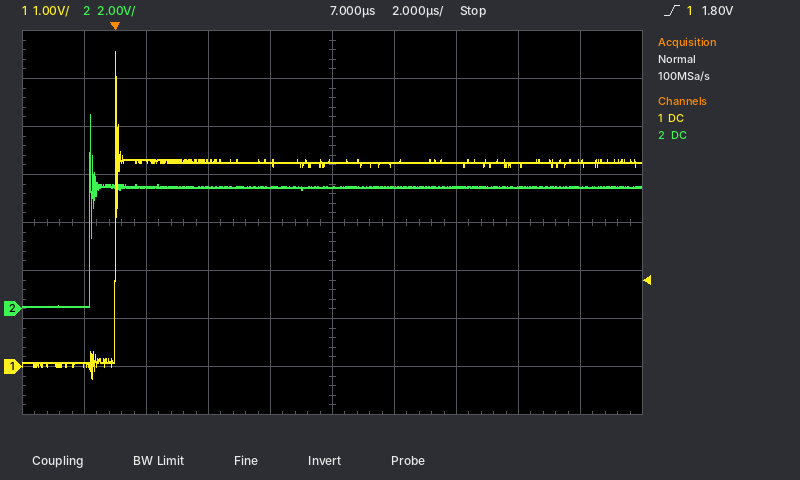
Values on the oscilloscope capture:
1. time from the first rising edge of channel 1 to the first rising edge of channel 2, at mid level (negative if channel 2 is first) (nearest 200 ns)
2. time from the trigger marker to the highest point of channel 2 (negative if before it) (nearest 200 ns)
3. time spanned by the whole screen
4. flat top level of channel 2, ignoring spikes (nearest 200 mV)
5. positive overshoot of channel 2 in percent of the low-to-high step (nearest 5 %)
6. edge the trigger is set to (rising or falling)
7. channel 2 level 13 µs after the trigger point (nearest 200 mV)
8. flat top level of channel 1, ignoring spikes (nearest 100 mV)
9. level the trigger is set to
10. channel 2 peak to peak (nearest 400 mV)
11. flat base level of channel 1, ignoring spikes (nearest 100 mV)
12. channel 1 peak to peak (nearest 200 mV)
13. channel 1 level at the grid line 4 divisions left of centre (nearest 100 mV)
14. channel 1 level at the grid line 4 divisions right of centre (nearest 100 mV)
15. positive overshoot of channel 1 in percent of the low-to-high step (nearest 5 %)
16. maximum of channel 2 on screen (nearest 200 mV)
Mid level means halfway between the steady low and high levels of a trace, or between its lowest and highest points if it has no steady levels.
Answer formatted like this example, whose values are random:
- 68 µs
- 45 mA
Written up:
- -800 ns
- -800 ns
- 20 µs
- 5.0 V
- 60 %
- rising
- 5.0 V
- 4.2 V
- 1.80 V
- 8.0 V
- 100 mV
- 6.8 V
- 0.0 V
- 4.3 V
- 55 %
- 8.0 V
